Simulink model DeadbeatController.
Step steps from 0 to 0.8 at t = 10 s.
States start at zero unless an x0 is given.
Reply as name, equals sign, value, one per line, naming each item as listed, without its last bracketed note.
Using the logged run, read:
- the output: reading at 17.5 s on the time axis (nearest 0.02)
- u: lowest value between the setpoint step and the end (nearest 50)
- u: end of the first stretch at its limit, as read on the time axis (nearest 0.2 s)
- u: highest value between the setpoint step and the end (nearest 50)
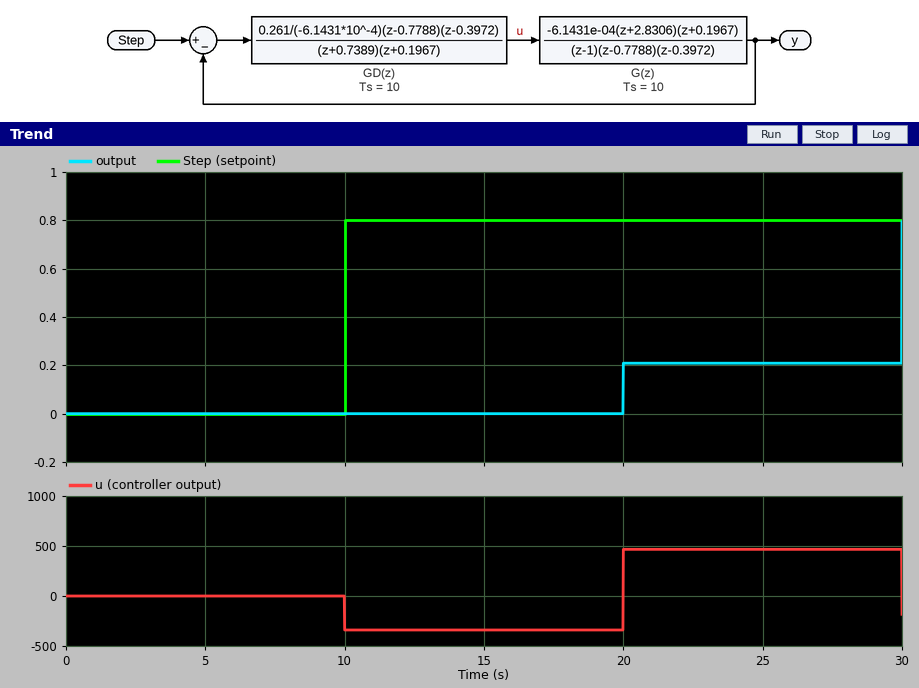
the output: reading at 17.5 s on the time axis = 0.00
u: lowest value between the setpoint step and the end = -350
u: end of the first stretch at its limit, as read on the time axis = 20.0 s
u: highest value between the setpoint step and the end = 450
